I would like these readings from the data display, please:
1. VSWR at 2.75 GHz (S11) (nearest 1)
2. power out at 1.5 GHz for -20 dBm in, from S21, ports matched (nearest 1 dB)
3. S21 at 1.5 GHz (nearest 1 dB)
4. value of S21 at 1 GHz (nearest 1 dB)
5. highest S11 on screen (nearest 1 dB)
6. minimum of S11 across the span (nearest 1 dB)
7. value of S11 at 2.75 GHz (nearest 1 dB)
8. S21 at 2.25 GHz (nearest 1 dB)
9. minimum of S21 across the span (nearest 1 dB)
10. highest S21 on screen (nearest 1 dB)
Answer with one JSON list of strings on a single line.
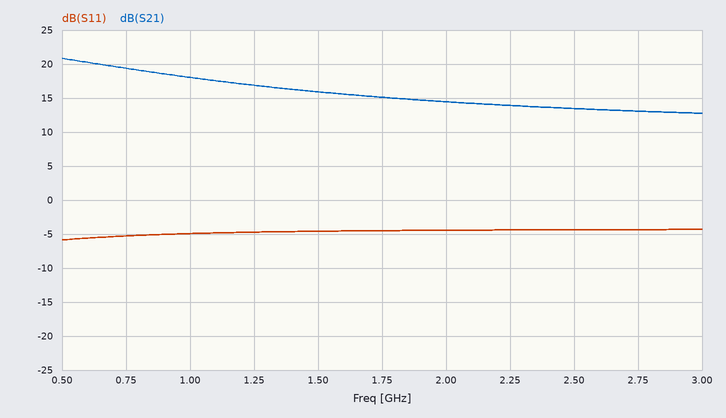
["4", "-4 dBm", "16 dB", "18 dB", "-4 dB", "-6 dB", "-4 dB", "14 dB", "13 dB", "21 dB"]
